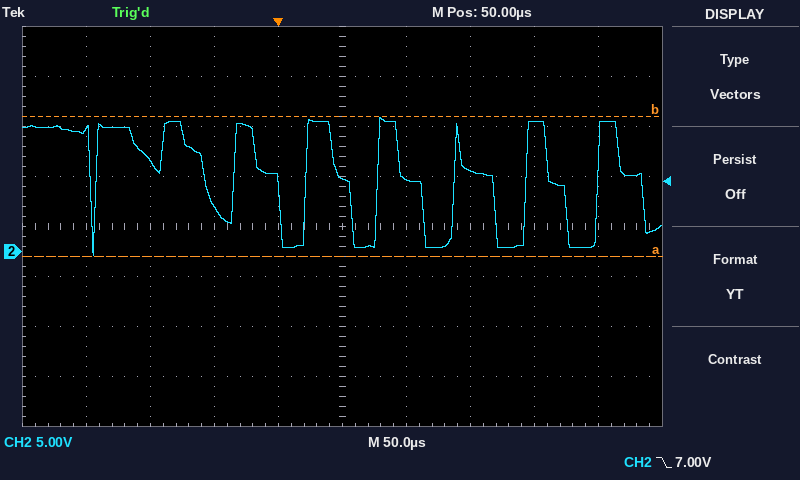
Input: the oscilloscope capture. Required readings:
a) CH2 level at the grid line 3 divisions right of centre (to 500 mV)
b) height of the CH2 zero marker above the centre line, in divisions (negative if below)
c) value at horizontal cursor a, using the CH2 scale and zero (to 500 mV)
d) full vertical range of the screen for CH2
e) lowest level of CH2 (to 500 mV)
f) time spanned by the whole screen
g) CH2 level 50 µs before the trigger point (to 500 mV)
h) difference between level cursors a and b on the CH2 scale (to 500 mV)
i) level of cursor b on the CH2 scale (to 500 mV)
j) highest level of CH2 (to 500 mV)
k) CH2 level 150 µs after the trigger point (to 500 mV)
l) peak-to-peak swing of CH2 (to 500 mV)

13.0 V
-0.5 div
-500 mV
40 V
-500 mV
500 µs
4.5 V
14.0 V
13.5 V
13.5 V
8.0 V
14.0 V
